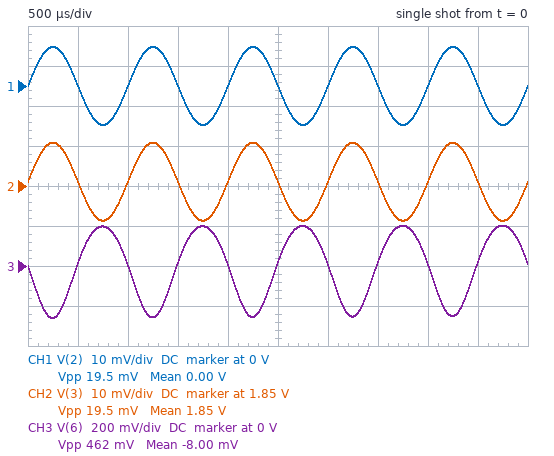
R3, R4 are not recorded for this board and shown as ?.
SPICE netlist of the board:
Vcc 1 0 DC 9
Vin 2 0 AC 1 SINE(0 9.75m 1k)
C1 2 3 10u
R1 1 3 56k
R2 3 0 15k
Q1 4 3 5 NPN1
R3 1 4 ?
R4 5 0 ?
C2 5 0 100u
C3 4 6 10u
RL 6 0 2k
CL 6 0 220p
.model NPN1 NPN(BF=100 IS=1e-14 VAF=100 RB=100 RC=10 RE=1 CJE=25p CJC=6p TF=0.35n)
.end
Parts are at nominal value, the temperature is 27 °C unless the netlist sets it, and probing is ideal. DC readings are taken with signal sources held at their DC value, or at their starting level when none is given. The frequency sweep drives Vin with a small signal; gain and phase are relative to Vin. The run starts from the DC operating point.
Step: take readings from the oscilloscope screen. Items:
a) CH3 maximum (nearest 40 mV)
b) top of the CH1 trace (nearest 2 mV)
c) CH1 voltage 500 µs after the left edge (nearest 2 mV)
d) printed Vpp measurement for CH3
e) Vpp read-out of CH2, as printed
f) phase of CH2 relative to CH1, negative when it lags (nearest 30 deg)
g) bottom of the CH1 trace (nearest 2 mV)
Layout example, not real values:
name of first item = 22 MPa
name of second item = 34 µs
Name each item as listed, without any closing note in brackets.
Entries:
CH3 maximum = 200 mV
top of the CH1 trace = 10 mV
CH1 voltage 500 µs after the left edge = 0 V
printed Vpp measurement for CH3 = 462 mV
Vpp read-out of CH2, as printed = 19.5 mV
phase of CH2 relative to CH1, negative when it lags = 0 deg
bottom of the CH1 trace = -10 mV
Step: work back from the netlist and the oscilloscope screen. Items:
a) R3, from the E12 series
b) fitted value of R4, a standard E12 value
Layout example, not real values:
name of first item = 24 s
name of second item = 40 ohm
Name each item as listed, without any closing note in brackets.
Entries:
R3, from the E12 series = 4.7 kΩ
fitted value of R4, a standard E12 value = 2.7 kΩ
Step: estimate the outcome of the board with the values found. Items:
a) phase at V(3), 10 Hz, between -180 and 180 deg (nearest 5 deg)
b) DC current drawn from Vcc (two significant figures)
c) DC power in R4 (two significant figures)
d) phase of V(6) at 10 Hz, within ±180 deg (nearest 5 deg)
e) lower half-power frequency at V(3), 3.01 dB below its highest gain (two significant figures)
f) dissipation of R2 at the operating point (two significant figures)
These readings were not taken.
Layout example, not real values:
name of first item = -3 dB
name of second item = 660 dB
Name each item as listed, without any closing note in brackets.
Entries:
phase at V(3), 10 Hz, between -180 and 180 deg = 10 deg
DC current drawn from Vcc = 570 µA
DC power in R4 = 550 µW
phase of V(6) at 10 Hz, within ±180 deg = -90 deg
lower half-power frequency at V(3), 3.01 dB below its highest gain = 1.6 Hz
dissipation of R2 at the operating point = 230 µW
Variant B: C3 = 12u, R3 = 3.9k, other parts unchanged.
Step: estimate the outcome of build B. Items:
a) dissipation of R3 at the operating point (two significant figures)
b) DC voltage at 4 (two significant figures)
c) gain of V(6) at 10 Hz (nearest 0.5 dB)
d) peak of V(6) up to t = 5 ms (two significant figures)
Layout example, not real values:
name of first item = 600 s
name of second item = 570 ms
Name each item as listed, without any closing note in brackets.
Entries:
dissipation of R3 at the operating point = 780 µW
DC voltage at 4 = 7.3 V
gain of V(6) at 10 Hz = 16.5 dB
peak of V(6) up to t = 5 ms = 190 mV
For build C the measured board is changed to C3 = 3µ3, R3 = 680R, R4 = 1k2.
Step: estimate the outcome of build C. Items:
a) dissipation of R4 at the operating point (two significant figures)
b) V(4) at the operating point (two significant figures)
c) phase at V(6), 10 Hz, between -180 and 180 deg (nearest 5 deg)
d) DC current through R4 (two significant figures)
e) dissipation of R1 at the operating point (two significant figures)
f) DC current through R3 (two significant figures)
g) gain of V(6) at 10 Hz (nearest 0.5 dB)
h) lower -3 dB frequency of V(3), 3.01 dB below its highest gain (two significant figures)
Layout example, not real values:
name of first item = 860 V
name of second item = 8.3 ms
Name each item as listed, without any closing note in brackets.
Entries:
dissipation of R4 at the operating point = 1.1 mW
V(4) at the operating point = 8.4 V
phase at V(6), 10 Hz, between -180 and 180 deg = -40 deg
DC current through R4 = 950 µA
dissipation of R1 at the operating point = 930 µW
DC current through R3 = 940 µA
gain of V(6) at 10 Hz = 2.5 dB
lower -3 dB frequency of V(3), 3.01 dB below its highest gain = 1.6 Hz
